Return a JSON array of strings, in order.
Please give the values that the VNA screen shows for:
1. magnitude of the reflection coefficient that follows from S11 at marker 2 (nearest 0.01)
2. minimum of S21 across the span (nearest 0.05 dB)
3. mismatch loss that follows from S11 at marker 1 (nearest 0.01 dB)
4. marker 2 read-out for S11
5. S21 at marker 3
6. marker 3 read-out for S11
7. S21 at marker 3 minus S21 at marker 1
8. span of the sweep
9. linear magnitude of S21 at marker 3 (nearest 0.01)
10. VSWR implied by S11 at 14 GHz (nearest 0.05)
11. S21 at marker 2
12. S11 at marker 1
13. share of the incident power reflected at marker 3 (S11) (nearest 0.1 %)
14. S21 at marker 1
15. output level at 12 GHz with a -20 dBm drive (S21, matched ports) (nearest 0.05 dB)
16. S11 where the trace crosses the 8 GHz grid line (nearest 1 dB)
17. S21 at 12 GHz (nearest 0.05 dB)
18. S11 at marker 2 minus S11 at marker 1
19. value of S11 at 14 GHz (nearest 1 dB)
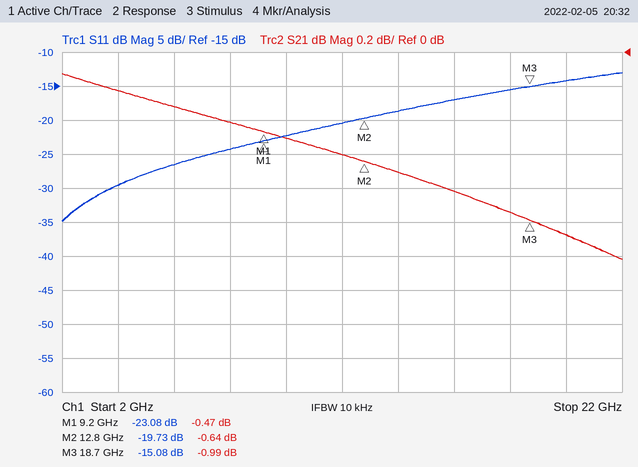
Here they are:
["0.10", "-1.20 dB", "0.02 dB", "-19.73 dB", "-0.99 dB", "-15.08 dB", "-0.52 dB", "20 GHz", "0.89", "1.25", "-0.64 dB", "-23.08 dB", "3.1 %", "-0.47 dB", "-20.60 dBm", "-24 dB", "-0.60 dB", "3.35 dB", "-19 dB"]
